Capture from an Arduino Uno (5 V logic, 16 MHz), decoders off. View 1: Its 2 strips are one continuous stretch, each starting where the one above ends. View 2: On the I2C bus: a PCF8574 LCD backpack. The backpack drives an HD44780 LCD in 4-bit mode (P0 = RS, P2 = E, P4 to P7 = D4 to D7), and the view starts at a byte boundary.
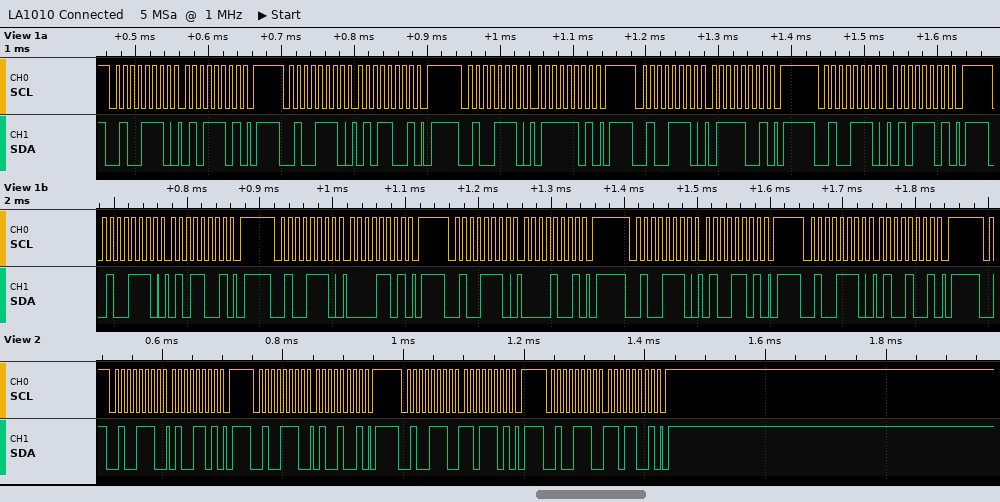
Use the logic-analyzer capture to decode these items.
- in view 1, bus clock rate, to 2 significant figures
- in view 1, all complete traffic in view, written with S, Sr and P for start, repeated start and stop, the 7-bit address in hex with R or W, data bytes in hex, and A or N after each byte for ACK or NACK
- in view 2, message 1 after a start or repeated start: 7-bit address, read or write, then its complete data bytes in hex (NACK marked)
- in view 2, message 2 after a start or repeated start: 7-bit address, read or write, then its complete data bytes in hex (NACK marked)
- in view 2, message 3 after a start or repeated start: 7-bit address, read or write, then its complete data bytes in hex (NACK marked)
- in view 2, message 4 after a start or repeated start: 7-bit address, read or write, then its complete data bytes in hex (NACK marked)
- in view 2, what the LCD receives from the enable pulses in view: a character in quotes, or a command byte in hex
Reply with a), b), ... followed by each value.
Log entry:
a) 100 kHz
b) S 27W A 5D A P S 27W A 59 A P S 27W A 7D A P S 27W A 79 A P S 27W A 5D A P S 27W A 59 A P S 27W A 0D A P S 27W A 09 A P S 27W A 4D A P S 27W A 49 A P
c) 0x27 write: 4D
d) 0x27 write: 49
e) 0x27 write: DD
f) 0x27 write: D9
g) 'M'
